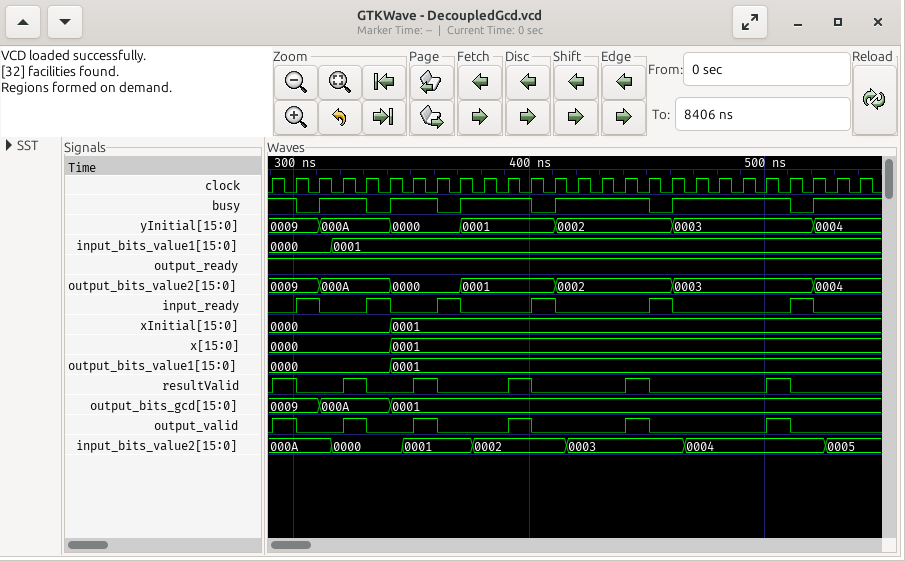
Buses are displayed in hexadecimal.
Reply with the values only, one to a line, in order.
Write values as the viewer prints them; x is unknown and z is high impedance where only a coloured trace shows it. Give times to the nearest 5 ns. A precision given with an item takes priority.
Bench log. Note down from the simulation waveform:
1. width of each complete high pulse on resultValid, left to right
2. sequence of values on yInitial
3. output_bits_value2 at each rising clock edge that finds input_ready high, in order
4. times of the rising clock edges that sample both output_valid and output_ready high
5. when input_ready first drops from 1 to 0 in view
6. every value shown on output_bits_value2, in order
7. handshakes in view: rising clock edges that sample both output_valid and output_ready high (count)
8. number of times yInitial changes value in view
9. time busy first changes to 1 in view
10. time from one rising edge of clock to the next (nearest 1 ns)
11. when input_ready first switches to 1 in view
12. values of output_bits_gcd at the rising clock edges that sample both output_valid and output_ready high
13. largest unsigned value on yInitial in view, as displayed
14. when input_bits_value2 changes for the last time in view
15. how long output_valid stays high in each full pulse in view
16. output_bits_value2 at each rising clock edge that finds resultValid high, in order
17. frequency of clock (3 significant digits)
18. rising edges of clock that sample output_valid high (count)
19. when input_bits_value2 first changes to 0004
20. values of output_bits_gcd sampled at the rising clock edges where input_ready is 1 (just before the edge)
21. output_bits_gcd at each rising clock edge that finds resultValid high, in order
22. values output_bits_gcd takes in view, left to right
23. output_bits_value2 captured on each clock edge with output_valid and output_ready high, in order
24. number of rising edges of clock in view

10 ns, 10 ns, 10 ns, 10 ns, 10 ns, 10 ns
0009, 000A, 0000, 0001, 0002, 0003, 0004
0009, 000A, 0000, 0001, 0002, 0003
300 ns, 330 ns, 360 ns, 400 ns, 450 ns, 510 ns
310 ns
0009, 000A, 0000, 0001, 0002, 0003, 0004
6
6
310 ns
10 ns
300 ns
0009, 000A, 0001, 0001, 0001, 0001
000A
525 ns
10 ns, 10 ns, 10 ns, 10 ns, 10 ns, 10 ns
0009, 000A, 0000, 0001, 0002, 0003
100 MHz
6
465 ns
0009, 000A, 0001, 0001, 0001, 0001
0009, 000A, 0001, 0001, 0001, 0001
0009, 000A, 0001
0009, 000A, 0000, 0001, 0002, 0003
26
